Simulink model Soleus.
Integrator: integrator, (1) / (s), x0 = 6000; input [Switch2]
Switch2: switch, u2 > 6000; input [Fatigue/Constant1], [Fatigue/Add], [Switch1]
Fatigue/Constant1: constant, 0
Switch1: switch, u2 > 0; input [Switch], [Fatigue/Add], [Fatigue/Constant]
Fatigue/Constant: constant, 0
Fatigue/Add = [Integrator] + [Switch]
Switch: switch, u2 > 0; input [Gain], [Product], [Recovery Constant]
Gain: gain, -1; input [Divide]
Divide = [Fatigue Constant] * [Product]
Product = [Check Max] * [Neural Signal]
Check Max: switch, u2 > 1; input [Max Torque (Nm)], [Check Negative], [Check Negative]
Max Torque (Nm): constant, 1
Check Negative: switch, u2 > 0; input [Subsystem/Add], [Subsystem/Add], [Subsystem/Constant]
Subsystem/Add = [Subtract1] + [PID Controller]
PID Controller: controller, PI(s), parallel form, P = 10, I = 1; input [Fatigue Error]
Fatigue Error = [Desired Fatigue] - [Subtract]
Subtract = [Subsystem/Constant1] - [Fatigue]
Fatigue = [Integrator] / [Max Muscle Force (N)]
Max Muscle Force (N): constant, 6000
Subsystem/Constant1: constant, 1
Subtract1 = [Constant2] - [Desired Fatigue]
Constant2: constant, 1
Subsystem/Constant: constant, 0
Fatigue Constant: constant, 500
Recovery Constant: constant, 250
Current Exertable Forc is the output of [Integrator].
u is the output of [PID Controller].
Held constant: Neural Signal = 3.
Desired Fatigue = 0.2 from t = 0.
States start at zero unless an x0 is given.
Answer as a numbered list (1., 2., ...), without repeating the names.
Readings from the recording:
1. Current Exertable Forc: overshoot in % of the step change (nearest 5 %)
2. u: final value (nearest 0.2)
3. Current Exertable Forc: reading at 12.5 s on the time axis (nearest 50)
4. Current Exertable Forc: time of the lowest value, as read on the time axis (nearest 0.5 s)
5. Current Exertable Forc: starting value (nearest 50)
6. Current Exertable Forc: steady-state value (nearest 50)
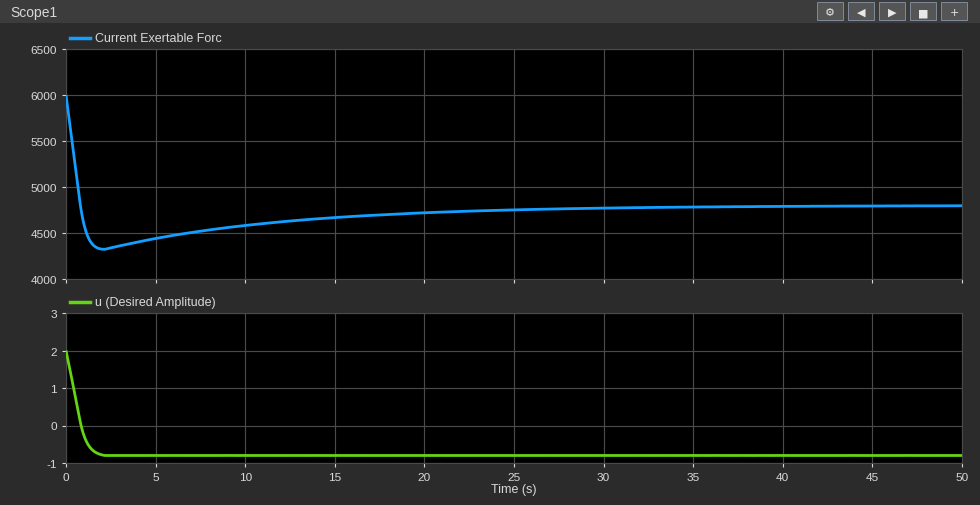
1. 40 %
2. -0.8
3. 4650
4. 2.0 s
5. 6000
6. 4800
